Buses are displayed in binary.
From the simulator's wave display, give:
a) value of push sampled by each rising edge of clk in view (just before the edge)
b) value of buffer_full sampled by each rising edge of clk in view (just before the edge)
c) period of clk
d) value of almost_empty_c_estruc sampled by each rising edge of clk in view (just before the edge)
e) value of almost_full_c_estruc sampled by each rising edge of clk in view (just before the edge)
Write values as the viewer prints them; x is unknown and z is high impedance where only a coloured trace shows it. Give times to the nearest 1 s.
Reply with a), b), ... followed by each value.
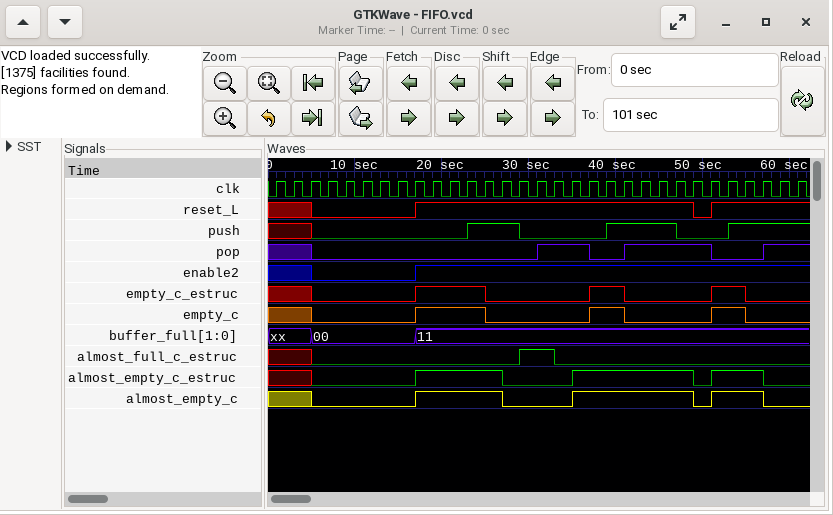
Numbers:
a) x x x 0 0 0 0 0 0 0 0 0 1 1 1 0 0 0 0 0 1 1 1 1 0 0 0 1 1 1 1
b) xx, xx, xx, 00, 00, 00, 00, 00, 00, 11, 11, 11, 11, 11, 11, 11, 11, 11, 11, 11, 11, 11, 11, 11, 11, 11, 11, 11, 11, 11, 11
c) 2 s
d) x x x 0 0 0 0 0 0 1 1 1 1 1 0 0 0 0 1 1 1 1 1 1 1 0 1 1 1 0 0
e) x x x 0 0 0 0 0 0 0 0 0 0 0 0 1 1 0 0 0 0 0 0 0 0 0 0 0 0 0 0
